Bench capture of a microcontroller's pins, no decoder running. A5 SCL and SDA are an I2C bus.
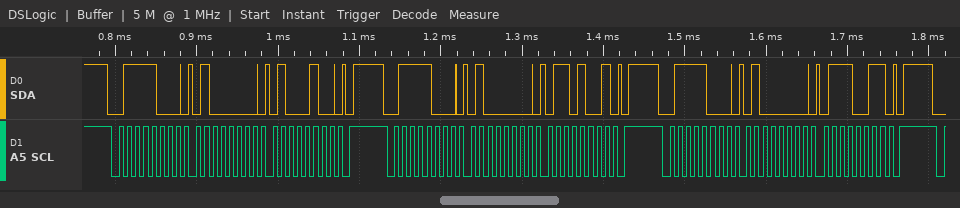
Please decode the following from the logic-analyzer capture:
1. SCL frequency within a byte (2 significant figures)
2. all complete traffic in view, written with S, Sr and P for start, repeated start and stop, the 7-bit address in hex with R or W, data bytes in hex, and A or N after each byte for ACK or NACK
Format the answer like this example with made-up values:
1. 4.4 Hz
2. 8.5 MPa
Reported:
1. 100 kHz
2. S 3CW A 40 A 44 A P S 3CW A 40 A 69 A P S 3CW A 40 A 73 A P
